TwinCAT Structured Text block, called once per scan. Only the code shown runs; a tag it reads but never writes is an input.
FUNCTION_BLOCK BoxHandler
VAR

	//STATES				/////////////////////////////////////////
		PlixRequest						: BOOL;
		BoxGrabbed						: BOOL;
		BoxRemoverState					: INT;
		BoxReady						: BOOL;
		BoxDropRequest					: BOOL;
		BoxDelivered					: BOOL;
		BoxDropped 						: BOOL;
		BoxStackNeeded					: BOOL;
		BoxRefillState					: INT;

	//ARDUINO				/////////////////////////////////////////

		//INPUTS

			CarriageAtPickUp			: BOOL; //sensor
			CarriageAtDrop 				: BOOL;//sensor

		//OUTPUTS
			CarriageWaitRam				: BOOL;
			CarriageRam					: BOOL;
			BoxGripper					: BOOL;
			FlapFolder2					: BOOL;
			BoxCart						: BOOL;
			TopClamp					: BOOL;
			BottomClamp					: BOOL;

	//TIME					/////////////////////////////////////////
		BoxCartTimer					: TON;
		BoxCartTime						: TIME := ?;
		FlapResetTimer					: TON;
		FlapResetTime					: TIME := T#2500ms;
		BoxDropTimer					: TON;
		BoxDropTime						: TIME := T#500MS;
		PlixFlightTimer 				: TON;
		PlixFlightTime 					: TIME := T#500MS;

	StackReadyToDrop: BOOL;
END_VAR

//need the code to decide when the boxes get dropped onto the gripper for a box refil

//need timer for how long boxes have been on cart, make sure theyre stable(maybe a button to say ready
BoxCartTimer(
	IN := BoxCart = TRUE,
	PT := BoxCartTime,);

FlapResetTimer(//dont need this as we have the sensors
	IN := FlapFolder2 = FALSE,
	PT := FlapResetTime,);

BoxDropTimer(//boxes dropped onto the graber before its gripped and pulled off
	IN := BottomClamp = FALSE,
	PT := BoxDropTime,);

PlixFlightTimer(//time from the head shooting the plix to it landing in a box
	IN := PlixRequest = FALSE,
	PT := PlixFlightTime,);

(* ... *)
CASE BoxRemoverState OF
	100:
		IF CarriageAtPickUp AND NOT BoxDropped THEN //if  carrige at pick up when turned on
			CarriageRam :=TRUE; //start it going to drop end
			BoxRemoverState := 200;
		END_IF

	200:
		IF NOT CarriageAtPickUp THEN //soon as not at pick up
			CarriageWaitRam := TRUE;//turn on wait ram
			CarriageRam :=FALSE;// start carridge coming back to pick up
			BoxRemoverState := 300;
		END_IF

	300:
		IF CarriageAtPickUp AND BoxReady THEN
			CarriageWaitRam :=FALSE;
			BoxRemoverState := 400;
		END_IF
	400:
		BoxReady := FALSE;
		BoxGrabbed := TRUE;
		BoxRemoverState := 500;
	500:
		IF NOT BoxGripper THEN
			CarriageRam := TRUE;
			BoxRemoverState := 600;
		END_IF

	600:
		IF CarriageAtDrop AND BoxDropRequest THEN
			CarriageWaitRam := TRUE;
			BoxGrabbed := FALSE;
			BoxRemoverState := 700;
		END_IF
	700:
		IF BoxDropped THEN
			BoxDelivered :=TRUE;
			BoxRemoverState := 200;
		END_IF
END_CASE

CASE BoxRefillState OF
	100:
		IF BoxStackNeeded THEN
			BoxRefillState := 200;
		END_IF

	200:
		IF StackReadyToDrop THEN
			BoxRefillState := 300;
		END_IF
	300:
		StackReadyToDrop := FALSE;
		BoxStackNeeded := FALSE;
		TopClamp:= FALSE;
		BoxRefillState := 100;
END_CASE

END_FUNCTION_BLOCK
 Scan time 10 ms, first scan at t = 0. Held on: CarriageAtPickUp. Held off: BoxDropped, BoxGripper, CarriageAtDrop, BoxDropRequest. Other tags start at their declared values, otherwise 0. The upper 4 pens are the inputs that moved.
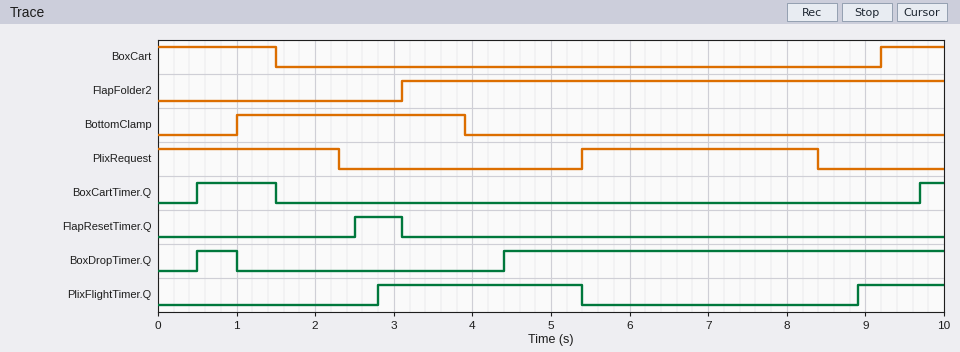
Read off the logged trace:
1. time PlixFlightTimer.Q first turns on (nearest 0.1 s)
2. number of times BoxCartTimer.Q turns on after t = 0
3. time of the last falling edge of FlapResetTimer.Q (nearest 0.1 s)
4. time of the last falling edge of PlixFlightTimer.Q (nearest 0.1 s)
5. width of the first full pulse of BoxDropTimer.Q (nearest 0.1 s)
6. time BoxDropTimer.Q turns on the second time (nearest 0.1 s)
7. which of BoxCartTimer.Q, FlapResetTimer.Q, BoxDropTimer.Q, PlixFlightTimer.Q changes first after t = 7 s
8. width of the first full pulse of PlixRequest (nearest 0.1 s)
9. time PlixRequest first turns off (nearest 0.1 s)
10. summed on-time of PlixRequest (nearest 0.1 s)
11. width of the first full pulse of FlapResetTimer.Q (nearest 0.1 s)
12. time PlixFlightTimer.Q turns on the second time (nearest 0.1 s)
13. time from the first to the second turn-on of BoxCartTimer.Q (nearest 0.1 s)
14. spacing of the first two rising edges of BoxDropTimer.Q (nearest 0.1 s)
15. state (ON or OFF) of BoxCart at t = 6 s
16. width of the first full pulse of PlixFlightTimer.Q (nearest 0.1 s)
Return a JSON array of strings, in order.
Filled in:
["2.8 s", "2", "3.1 s", "5.4 s", "0.5 s", "4.4 s", "PlixFlightTimer.Q", "3.0 s", "2.3 s", "5.3 s", "0.6 s", "8.9 s", "9.2 s", "3.9 s", "OFF", "2.6 s"]
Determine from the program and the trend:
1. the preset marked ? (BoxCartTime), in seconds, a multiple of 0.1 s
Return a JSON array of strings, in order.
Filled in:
["0.5 s"]
